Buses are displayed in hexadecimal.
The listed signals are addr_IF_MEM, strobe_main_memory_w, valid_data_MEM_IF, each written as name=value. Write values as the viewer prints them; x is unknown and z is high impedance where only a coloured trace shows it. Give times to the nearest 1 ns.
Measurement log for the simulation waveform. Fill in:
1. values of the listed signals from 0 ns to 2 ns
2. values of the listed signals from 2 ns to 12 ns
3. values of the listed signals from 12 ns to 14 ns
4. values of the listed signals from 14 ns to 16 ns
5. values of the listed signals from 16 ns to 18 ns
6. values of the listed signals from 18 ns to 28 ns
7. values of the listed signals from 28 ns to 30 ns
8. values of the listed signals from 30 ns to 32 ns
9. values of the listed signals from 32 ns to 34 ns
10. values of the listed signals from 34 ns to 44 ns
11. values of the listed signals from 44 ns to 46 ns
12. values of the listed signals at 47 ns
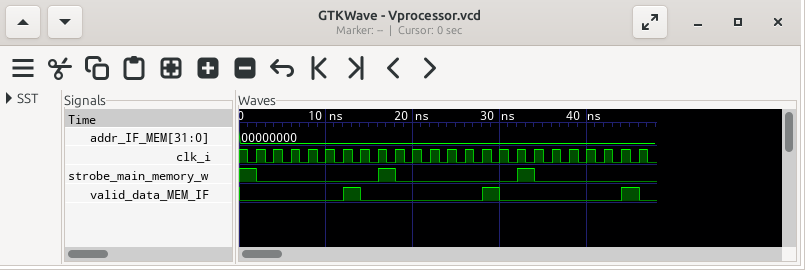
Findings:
addr_IF_MEM=00000000, strobe_main_memory_w=1, valid_data_MEM_IF=0
addr_IF_MEM=00000000, strobe_main_memory_w=0, valid_data_MEM_IF=0
addr_IF_MEM=00000000, strobe_main_memory_w=0, valid_data_MEM_IF=1
addr_IF_MEM=00000000, strobe_main_memory_w=0, valid_data_MEM_IF=0
addr_IF_MEM=00000000, strobe_main_memory_w=1, valid_data_MEM_IF=0
addr_IF_MEM=00000000, strobe_main_memory_w=0, valid_data_MEM_IF=0
addr_IF_MEM=00000000, strobe_main_memory_w=0, valid_data_MEM_IF=1
addr_IF_MEM=00000000, strobe_main_memory_w=0, valid_data_MEM_IF=0
addr_IF_MEM=00000000, strobe_main_memory_w=1, valid_data_MEM_IF=0
addr_IF_MEM=00000000, strobe_main_memory_w=0, valid_data_MEM_IF=0
addr_IF_MEM=00000000, strobe_main_memory_w=0, valid_data_MEM_IF=1
addr_IF_MEM=00000000, strobe_main_memory_w=0, valid_data_MEM_IF=0
